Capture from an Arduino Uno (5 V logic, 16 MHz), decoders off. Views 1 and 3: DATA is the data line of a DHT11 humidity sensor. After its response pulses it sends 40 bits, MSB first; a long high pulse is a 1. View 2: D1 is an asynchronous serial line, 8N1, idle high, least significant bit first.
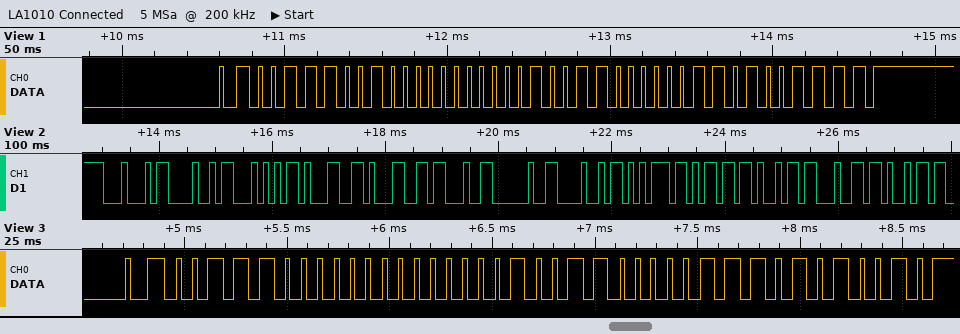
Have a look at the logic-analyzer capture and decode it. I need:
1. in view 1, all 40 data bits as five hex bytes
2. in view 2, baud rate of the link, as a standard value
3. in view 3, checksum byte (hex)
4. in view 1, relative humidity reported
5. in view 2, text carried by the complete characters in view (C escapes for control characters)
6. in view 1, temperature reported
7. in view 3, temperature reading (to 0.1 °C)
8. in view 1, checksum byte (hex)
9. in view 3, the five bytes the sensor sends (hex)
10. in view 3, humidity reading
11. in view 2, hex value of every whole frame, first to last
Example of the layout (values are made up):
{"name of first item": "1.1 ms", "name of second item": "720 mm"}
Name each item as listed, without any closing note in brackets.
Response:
{"in view 1, all 40 data bits as five hex bytes": "39 00 13 03 4F", "in view 2, baud rate of the link, as a standard value": "9600 baud", "in view 3, checksum byte": "0x52", "in view 1, relative humidity reported": "57 %", "in view 2, text carried by the complete characters in view": "\"DHT11# Humidi\"", "in view 1, temperature reported": "19.3 °C", "in view 3, temperature reading": "19.7 °C", "in view 1, checksum byte": "0x4F", "in view 3, the five bytes the sensor sends": "38 00 13 07 52", "in view 3, humidity reading": "56 %", "in view 2, hex value of every whole frame, first to last": "44 48 54 31 31 23 20 48 75 6D 69 64 69"}
